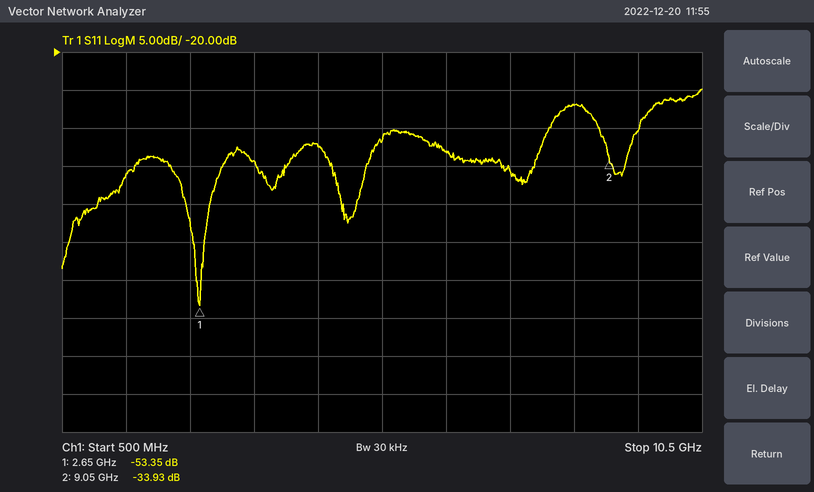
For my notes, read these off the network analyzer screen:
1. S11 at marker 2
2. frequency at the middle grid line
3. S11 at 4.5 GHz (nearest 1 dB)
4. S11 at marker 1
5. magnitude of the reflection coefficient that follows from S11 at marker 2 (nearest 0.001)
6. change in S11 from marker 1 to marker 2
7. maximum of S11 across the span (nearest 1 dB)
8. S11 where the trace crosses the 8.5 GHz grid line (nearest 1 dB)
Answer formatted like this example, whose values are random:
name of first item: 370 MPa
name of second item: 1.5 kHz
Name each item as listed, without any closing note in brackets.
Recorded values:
S11 at marker 2: -33.93 dB
frequency at the middle grid line: 5.5 GHz
S11 at 4.5 GHz: -32 dB
S11 at marker 1: -53.35 dB
magnitude of the reflection coefficient that follows from S11 at marker 2: 0.020
change in S11 from marker 1 to marker 2: 19.42 dB
maximum of S11 across the span: -25 dB
S11 where the trace crosses the 8.5 GHz grid line: -27 dB
